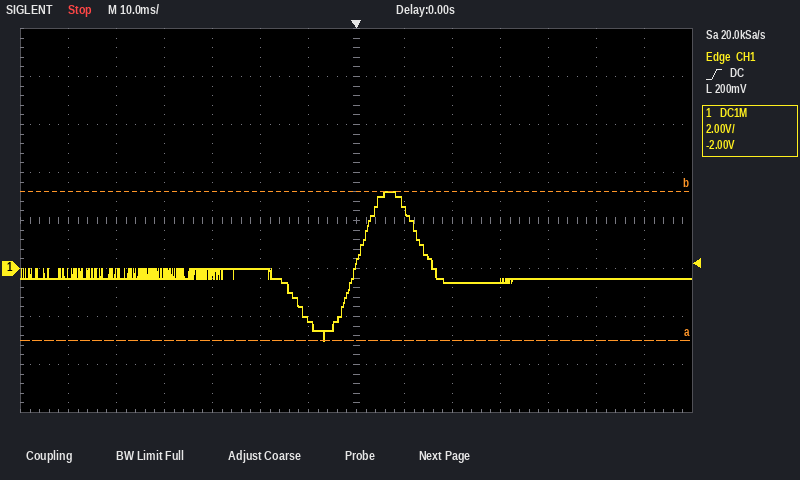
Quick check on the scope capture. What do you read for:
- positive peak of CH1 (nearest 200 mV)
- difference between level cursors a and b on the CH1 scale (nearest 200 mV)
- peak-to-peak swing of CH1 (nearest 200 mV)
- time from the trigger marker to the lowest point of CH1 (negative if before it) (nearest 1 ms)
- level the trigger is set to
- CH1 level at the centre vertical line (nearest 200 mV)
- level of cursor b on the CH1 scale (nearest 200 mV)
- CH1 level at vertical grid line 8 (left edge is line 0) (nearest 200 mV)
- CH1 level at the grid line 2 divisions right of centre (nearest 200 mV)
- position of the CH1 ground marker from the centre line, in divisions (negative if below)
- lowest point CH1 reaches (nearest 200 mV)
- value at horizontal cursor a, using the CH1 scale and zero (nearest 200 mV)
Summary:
3.2 V
6.2 V
6.2 V
-7 ms
200 mV
200 mV
3.2 V
2.4 V
-600 mV
-1.0 div
-3.0 V
-3.0 V
